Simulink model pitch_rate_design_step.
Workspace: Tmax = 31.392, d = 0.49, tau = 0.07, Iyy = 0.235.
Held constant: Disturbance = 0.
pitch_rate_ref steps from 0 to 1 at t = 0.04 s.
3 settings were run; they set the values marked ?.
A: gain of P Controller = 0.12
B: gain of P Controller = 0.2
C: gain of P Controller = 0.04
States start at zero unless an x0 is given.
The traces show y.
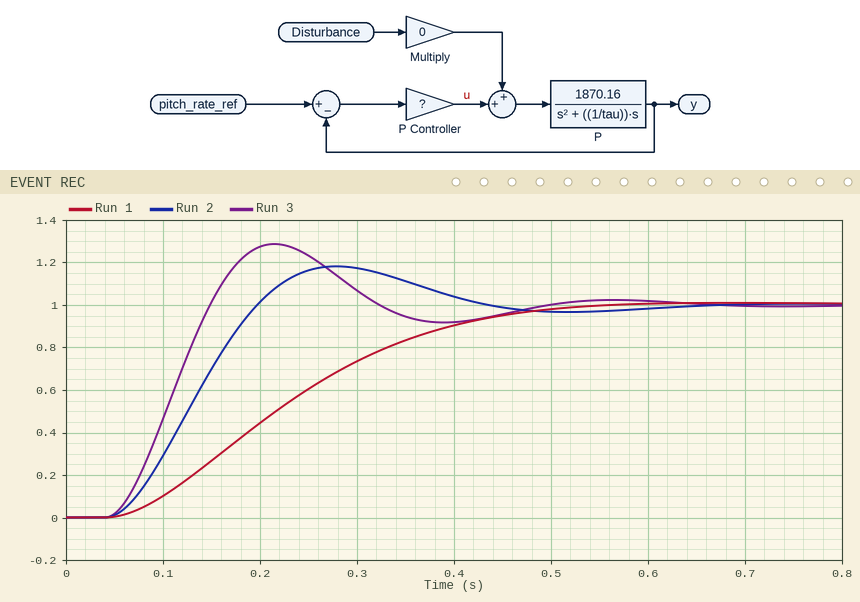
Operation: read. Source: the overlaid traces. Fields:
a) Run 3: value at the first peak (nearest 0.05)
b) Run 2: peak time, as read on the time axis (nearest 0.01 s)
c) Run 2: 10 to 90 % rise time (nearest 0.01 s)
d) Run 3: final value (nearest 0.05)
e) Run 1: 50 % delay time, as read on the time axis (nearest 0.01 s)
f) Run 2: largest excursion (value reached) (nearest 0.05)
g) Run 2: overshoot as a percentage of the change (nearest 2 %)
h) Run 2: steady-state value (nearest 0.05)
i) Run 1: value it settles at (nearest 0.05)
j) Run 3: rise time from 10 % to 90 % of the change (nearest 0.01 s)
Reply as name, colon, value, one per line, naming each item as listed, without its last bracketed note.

Run 3: value at the first peak: 1.30
Run 2: peak time, as read on the time axis: 0.28 s
Run 2: 10 to 90 % rise time: 0.11 s
Run 3: final value: 1.00
Run 1: 50 % delay time, as read on the time axis: 0.22 s
Run 2: largest excursion (value reached): 1.20
Run 2: overshoot as a percentage of the change: 18 %
Run 2: steady-state value: 1.00
Run 1: value it settles at: 1.00
Run 3: rise time from 10 % to 90 % of the change: 0.07 s
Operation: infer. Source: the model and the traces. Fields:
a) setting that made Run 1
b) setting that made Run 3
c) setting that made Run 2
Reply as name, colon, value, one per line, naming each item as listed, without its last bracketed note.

setting that made Run 1: C
setting that made Run 3: B
setting that made Run 2: A
